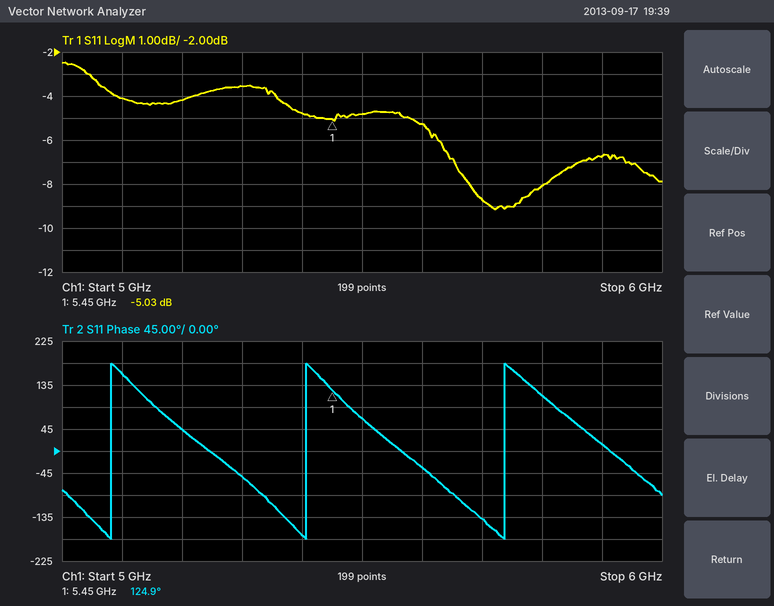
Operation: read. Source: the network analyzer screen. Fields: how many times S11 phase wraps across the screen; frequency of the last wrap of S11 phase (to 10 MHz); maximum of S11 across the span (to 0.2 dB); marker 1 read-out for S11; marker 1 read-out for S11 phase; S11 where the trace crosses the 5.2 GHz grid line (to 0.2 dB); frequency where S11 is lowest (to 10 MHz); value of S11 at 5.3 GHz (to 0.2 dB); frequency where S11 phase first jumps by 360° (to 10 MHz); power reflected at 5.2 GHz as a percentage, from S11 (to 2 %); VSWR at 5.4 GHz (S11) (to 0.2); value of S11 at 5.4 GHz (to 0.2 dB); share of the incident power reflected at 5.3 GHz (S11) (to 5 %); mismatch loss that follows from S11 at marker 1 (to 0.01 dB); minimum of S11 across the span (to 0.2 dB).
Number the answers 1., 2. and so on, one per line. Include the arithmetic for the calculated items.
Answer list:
1. 3
2. 5.74 GHz
3. -2.4 dB
4. -5.03 dB
5. 124.9°
6. -4.2 dB
7. 5.72 GHz
8. -3.6 dB
9. 5.08 GHz
10. 10^(-4.2/10) ≈ 38 %
11. |Γ| = 10^(-4.8/20) = 0.5754; VSWR = (1 + 0.5754)/(1 − 0.5754) ≈ 3.71, so 3.8 to the nearest 0.2
12. -4.8 dB
13. 10^(-3.6/10) ≈ 43.7 %, so 45 % to the nearest 5 %
14. −10 log10(1 − 10^(-5.03/10)) ≈ 1.64 dB
15. -9.2 dB
